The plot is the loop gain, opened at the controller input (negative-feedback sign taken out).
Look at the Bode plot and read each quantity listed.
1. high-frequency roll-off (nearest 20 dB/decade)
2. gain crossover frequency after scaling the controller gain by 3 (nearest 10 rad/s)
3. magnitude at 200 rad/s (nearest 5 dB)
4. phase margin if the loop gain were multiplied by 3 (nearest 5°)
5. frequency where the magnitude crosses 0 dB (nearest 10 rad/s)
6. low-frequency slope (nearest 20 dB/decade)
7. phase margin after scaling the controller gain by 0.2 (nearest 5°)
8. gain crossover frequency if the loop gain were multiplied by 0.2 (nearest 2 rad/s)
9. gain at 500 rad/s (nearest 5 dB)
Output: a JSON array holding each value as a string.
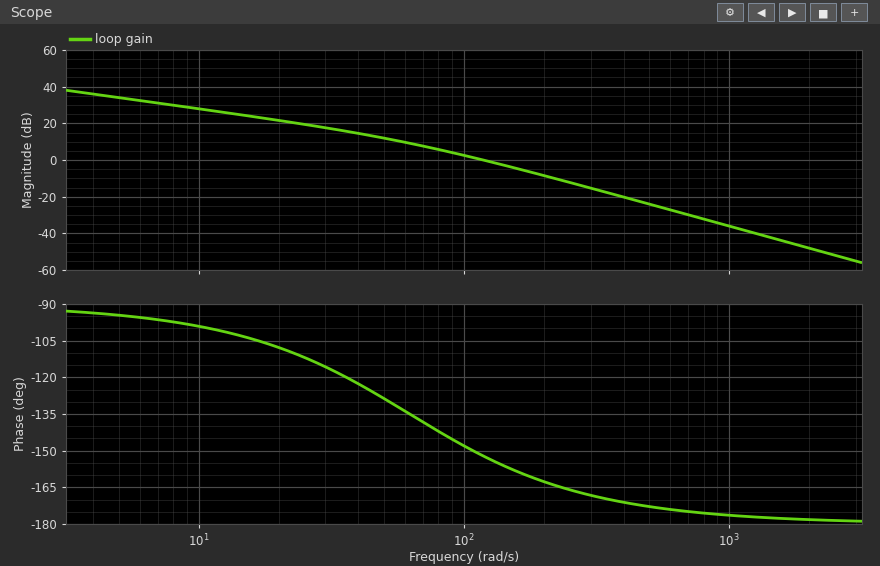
["-40 dB/decade", "210 rad/s", "-10 dB", "15°", "120 rad/s", "-20 dB/decade", "55°", "42 rad/s", "-25 dB"]
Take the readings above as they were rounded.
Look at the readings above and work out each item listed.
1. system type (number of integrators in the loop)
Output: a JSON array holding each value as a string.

["1"]
